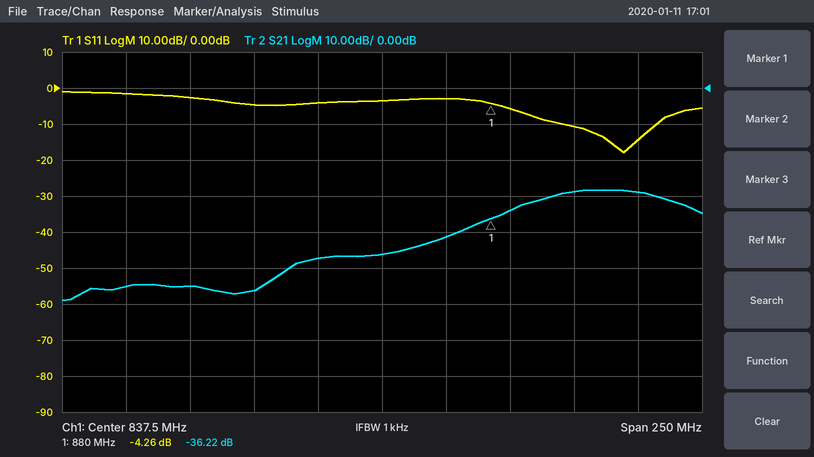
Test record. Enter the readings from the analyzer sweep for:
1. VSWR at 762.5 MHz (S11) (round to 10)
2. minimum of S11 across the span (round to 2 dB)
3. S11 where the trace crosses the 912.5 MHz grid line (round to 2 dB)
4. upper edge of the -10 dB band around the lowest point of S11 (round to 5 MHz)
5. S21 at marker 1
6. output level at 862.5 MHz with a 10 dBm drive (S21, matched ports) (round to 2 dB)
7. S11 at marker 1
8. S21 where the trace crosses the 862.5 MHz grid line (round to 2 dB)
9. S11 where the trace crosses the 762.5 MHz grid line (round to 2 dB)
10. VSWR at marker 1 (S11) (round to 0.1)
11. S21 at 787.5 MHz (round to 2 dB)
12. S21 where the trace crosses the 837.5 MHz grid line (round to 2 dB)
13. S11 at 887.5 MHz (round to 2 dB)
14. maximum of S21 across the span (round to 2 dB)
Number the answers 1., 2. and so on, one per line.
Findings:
1. 10
2. -18 dB
3. -10 dB
4. 945 MHz
5. -36.22 dB
6. -32 dBm
7. -4.26 dB
8. -42 dB
9. -2 dB
10. 4.2
11. -56 dB
12. -46 dB
13. -6 dB
14. -28 dB
